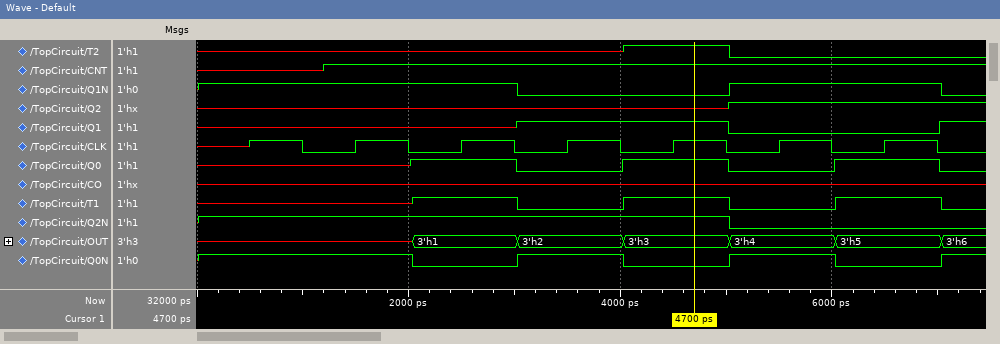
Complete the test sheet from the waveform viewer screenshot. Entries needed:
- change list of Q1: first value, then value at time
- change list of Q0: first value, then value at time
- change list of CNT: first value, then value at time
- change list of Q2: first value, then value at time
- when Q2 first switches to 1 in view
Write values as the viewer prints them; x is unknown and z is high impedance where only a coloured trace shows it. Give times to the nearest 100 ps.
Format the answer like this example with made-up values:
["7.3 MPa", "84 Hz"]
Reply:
["x, 1 at 3000 ps, 0 at 5000 ps, 1 at 7000 ps", "x, 1 at 2000 ps, 0 at 3000 ps, 1 at 4000 ps, 0 at 5000 ps, 1 at 6000 ps, 0 at 7000 ps", "x, 1 at 1200 ps", "x, 1 at 5000 ps", "5000 ps"]
